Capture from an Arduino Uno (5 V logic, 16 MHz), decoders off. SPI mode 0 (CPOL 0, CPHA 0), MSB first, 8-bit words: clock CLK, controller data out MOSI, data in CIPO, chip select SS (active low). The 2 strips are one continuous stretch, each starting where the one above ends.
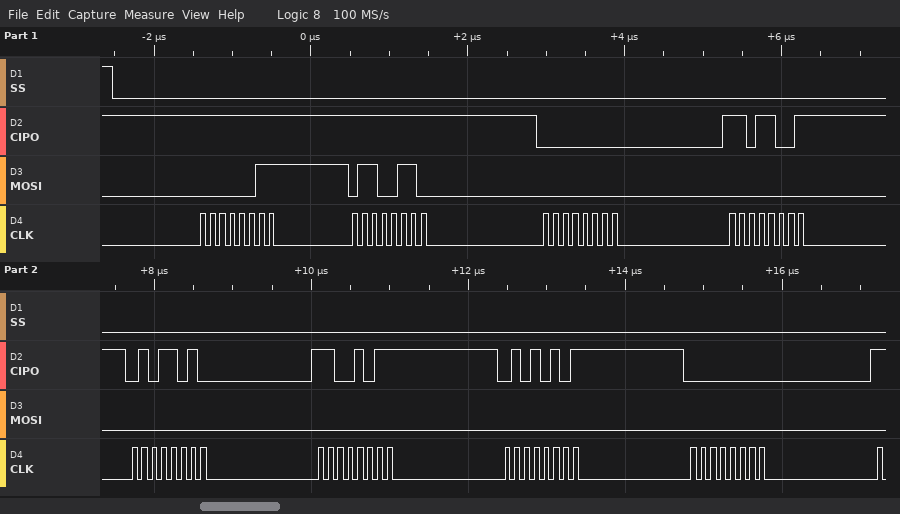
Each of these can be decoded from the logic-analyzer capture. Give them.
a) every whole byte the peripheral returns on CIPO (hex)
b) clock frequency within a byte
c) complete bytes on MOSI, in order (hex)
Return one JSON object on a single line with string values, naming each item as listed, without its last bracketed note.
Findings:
{"every whole byte the peripheral returns on CIPO": "FF FF 00 D9 5A CB 55 00", "clock frequency within a byte": "8 MHz", "complete bytes on MOSI, in order": "03 66 00 00 00 00 00 00"}
